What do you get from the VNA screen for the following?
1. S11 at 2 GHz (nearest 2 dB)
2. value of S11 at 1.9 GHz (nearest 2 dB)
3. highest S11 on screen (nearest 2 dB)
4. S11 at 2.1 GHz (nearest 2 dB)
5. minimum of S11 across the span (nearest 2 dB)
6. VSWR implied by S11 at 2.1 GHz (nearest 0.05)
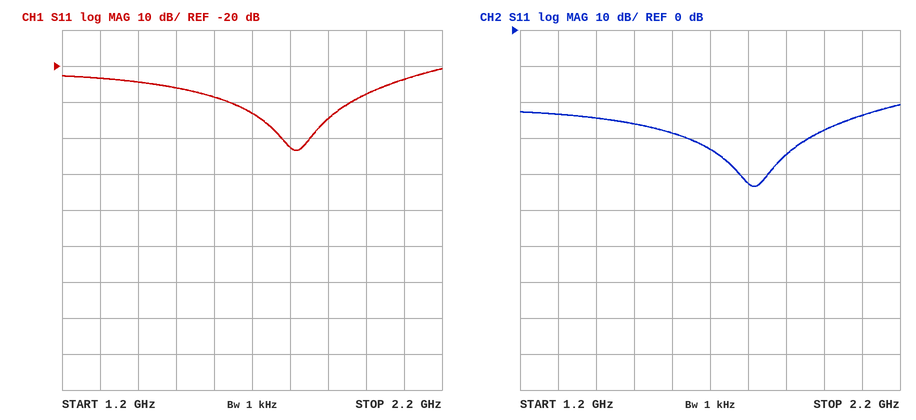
-28 dB
-34 dB
-20 dB
-24 dB
-44 dB
1.15
